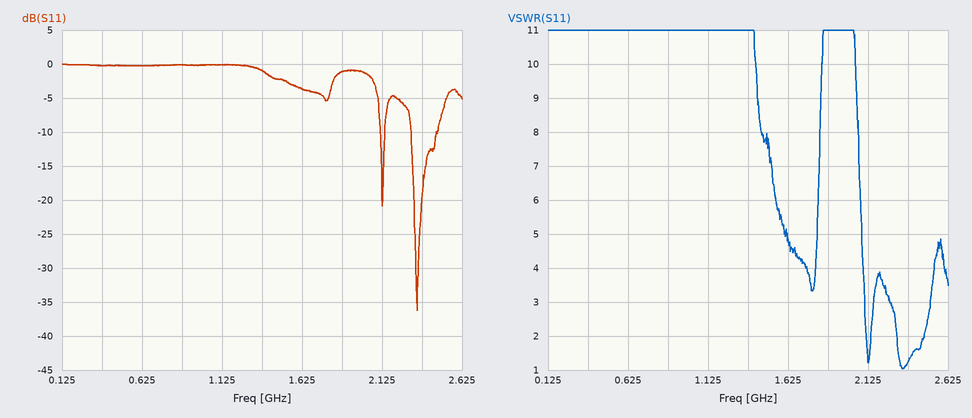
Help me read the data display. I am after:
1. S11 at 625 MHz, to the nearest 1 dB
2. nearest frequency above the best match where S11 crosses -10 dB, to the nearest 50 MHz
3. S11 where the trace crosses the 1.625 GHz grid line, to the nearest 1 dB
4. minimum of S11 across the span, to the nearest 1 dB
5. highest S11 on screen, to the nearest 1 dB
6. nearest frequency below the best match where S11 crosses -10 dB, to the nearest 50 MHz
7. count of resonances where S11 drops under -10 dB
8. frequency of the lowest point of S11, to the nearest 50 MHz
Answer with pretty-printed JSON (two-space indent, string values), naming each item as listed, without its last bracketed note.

{
  "S11 at 625 MHz, to the nearest 1 dB": "0 dB",
  "nearest frequency above the best match where S11 crosses -10 dB, to the nearest 50 MHz": "2.45 GHz",
  "S11 where the trace crosses the 1.625 GHz grid line, to the nearest 1 dB": "-4 dB",
  "minimum of S11 across the span, to the nearest 1 dB": "-36 dB",
  "highest S11 on screen, to the nearest 1 dB": "0 dB",
  "nearest frequency below the best match where S11 crosses -10 dB, to the nearest 50 MHz": "2.30 GHz",
  "count of resonances where S11 drops under -10 dB": "2",
  "frequency of the lowest point of S11, to the nearest 50 MHz": "2.35 GHz"
}
